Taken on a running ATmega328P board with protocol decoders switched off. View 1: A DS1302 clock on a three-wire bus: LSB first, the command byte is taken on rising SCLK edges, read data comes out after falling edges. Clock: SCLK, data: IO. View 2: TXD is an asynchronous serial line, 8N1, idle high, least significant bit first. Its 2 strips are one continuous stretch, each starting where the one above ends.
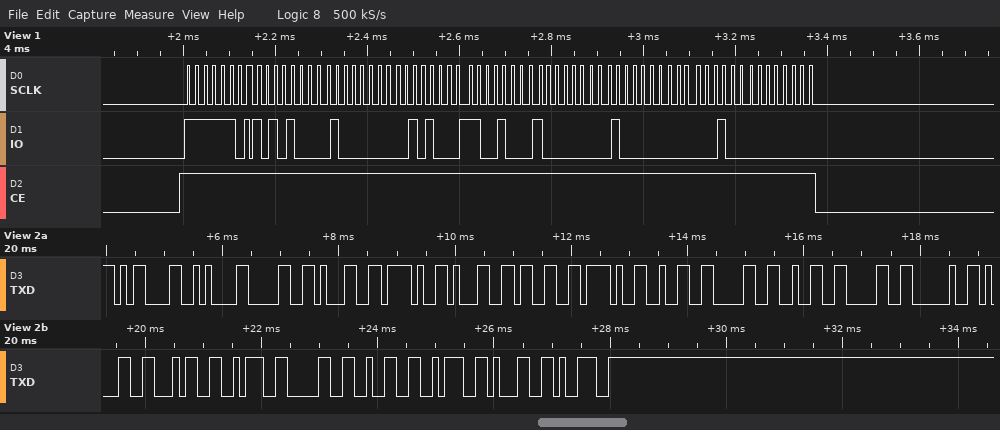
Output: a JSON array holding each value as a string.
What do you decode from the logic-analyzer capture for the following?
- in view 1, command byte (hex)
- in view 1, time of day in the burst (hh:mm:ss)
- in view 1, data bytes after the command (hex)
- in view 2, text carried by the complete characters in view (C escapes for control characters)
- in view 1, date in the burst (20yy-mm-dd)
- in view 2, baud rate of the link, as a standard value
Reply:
["0xBF", "14:02:15", "15 02 14 13 01 02 20 00", "\"\\r\\n01/13/2020 14:02:19\"", "2020-01-13", "9600 baud"]
